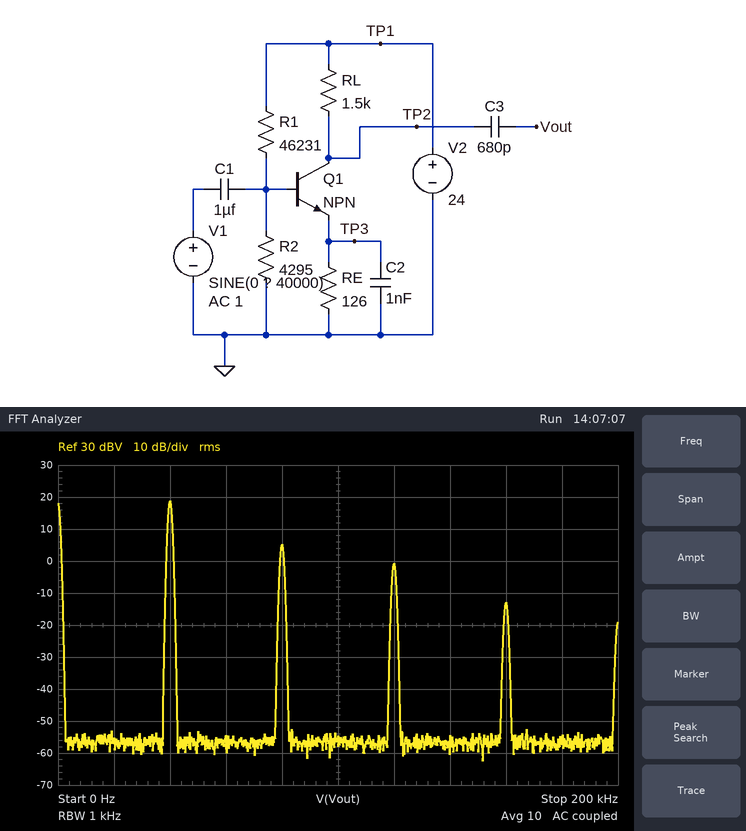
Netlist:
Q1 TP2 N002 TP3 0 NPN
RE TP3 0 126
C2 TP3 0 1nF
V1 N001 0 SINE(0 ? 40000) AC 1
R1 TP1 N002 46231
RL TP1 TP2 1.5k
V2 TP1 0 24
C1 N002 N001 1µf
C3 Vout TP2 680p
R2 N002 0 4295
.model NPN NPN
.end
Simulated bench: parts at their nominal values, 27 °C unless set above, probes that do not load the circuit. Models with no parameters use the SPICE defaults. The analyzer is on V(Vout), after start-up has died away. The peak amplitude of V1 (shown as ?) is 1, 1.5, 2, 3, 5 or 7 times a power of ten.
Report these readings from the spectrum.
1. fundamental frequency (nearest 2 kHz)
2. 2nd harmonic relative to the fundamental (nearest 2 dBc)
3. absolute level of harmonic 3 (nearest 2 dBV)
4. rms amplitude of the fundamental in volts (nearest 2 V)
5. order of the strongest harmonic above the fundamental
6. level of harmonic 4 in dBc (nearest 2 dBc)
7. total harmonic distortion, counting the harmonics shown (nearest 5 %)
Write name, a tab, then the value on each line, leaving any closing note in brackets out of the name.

fundamental frequency	40 kHz
2nd harmonic relative to the fundamental	-14 dBc
absolute level of harmonic 3	0 dBV
rms amplitude of the fundamental in volts	8 V
order of the strongest harmonic above the fundamental	2
level of harmonic 4 in dBc	-32 dBc
total harmonic distortion, counting the harmonics shown	25 %
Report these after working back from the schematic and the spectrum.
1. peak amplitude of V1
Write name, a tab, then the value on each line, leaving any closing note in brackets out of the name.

peak amplitude of V1	1.5 V
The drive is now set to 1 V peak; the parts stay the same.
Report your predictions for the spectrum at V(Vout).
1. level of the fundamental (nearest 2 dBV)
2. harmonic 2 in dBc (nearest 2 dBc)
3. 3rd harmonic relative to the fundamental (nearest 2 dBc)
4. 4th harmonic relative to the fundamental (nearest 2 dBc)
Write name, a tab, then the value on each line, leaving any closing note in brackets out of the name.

level of the fundamental	18 dBV
harmonic 2 in dBc	-34 dBc
3rd harmonic relative to the fundamental	-38 dBc
4th harmonic relative to the fundamental	-46 dBc
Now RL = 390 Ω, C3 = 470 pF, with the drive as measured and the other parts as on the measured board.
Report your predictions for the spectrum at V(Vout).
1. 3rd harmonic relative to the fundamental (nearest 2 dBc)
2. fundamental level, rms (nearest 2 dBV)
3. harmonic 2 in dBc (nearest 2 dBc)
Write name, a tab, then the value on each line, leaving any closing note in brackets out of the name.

3rd harmonic relative to the fundamental	-24 dBc
fundamental level, rms	8 dBV
harmonic 2 in dBc	-18 dBc
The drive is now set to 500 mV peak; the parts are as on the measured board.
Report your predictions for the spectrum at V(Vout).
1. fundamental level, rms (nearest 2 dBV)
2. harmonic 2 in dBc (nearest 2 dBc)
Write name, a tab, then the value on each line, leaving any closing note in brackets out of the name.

fundamental level, rms	12 dBV
harmonic 2 in dBc	-48 dBc
